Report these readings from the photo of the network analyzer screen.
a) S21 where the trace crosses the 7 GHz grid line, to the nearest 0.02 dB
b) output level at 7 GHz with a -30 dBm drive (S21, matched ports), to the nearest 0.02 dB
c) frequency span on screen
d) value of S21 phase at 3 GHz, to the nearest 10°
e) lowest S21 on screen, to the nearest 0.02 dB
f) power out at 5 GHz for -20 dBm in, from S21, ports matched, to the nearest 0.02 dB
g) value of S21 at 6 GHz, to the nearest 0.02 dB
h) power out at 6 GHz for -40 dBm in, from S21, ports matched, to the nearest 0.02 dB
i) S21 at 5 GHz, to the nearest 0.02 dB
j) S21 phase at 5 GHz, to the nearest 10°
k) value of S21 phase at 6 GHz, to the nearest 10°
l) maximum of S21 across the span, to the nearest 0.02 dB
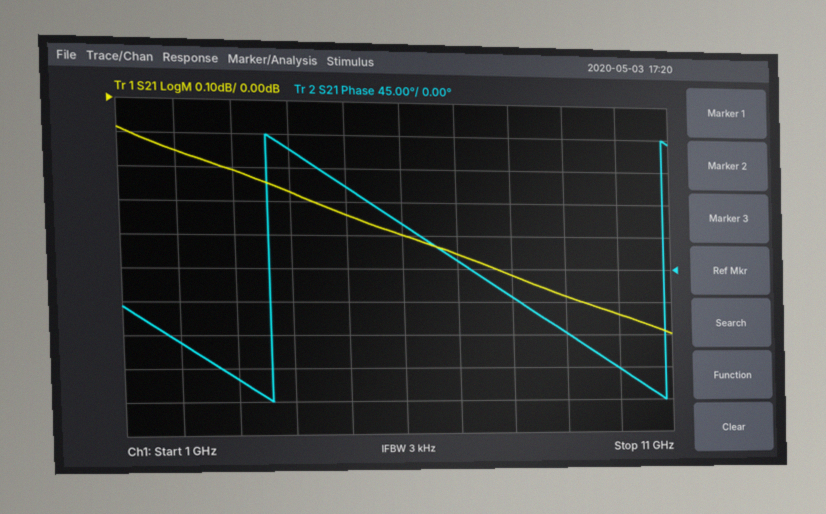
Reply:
-0.46 dB
-30.46 dBm
10 GHz
-150°
-0.70 dB
-20.34 dBm
-0.40 dB
-40.40 dBm
-0.34 dB
110°
60°
-0.08 dB
